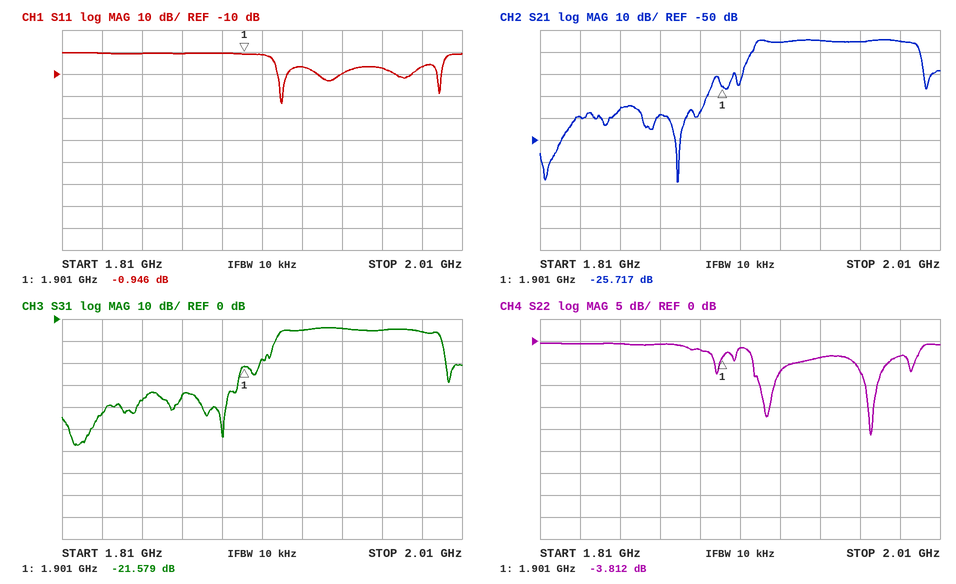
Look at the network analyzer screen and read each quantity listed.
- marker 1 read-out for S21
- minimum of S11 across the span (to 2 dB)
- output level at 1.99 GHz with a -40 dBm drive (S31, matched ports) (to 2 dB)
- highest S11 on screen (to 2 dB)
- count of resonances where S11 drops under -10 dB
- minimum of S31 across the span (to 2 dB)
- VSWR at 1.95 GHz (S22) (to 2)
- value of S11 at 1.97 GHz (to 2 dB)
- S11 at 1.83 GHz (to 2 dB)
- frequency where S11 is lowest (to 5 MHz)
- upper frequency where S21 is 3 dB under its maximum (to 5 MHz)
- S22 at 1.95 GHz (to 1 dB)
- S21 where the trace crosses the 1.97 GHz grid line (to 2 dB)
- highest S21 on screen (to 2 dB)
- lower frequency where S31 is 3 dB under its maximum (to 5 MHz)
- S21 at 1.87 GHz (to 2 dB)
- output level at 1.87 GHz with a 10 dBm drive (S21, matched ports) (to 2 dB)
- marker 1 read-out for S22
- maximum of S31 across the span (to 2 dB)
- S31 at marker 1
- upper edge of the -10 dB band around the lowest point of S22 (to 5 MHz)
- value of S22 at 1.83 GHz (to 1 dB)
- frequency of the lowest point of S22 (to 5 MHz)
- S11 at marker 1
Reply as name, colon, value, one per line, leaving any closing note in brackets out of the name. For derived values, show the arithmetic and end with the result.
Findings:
marker 1 read-out for S21: -25.717 dB
minimum of S11 across the span: -24 dB
output level at 1.99 GHz with a -40 dBm drive (S31, matched ports): -40 dBm + (-6 dB) = -46 dBm
highest S11 on screen: 0 dB
count of resonances where S11 drops under -10 dB: 4
minimum of S31 across the span: -58 dB
VSWR at 1.95 GHz (S22): |Γ| = 10^(-4/20) = 0.6310; VSWR = (1 + 0.6310)/(1 − 0.6310) ≈ 4
value of S11 at 1.97 GHz: -8 dB
S11 at 1.83 GHz: 0 dB
frequency where S11 is lowest: 1.920 GHz
upper frequency where S21 is 3 dB under its maximum: 2.000 GHz
S22 at 1.95 GHz: -4 dB
S21 where the trace crosses the 1.97 GHz grid line: -6 dB
highest S21 on screen: -4 dB
lower frequency where S31 is 3 dB under its maximum: 1.920 GHz
S21 at 1.87 GHz: -38 dB
output level at 1.87 GHz with a 10 dBm drive (S21, matched ports): 10 dBm + (-38 dB) = -28 dBm
marker 1 read-out for S22: -3.812 dB
maximum of S31 across the span: -4 dB
S31 at marker 1: -21.579 dB
upper edge of the -10 dB band around the lowest point of S22: 1.980 GHz
value of S22 at 1.83 GHz: -1 dB
frequency of the lowest point of S22: 1.975 GHz
S11 at marker 1: -0.946 dB
